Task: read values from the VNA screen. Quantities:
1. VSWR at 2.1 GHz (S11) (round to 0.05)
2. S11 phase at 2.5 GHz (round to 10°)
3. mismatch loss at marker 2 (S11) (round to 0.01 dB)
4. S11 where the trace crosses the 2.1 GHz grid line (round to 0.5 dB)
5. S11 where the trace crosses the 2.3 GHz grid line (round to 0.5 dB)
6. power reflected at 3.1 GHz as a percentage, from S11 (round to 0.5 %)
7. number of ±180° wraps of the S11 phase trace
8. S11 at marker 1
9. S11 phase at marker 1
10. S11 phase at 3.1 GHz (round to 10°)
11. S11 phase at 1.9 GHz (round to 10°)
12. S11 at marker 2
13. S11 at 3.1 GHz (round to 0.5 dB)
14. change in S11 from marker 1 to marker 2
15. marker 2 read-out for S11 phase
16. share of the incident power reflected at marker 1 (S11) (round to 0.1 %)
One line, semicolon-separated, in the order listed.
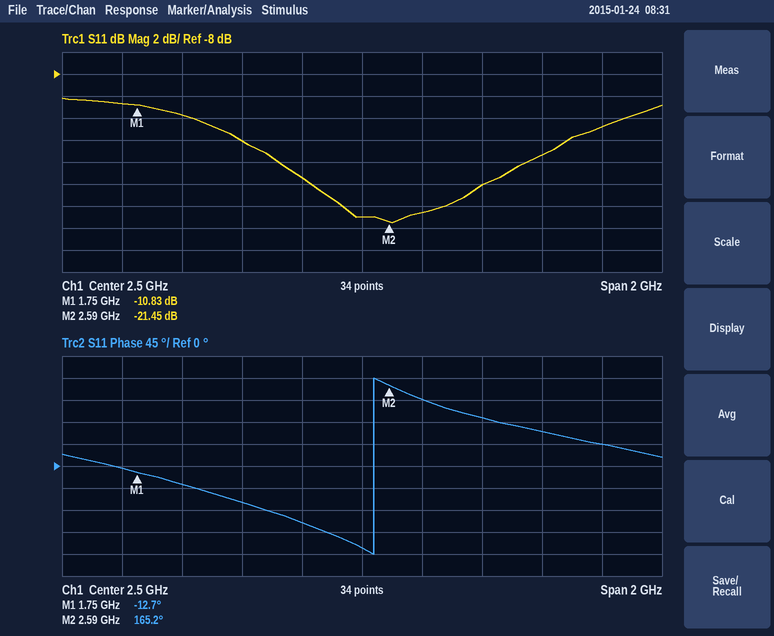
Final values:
1.50; -170°; 0.03 dB; -14.0 dB; -17.5 dB; 3.0 %; 1; -10.83 dB; -12.7°; 70°; -40°; -21.45 dB; -15.5 dB; -10.62 dB; 165.2°; 8.3 %
